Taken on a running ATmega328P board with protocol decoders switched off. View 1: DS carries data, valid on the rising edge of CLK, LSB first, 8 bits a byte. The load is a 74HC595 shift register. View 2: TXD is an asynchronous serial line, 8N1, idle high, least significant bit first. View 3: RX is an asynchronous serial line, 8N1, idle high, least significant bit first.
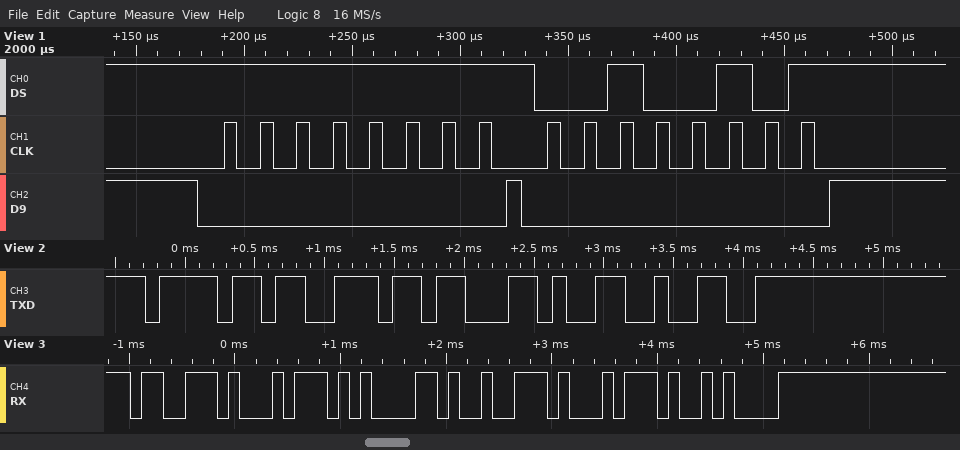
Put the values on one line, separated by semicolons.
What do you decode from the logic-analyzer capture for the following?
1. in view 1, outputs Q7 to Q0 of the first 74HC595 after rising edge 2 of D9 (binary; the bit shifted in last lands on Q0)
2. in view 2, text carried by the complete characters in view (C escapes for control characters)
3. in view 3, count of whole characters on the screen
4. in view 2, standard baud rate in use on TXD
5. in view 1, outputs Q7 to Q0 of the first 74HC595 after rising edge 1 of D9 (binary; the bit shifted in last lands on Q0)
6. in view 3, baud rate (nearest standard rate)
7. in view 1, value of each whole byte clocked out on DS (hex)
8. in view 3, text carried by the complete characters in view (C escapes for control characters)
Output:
00100101; "on,2"; 6; 9600 baud; 11111111; 9600 baud; FF A4; "start\n"
